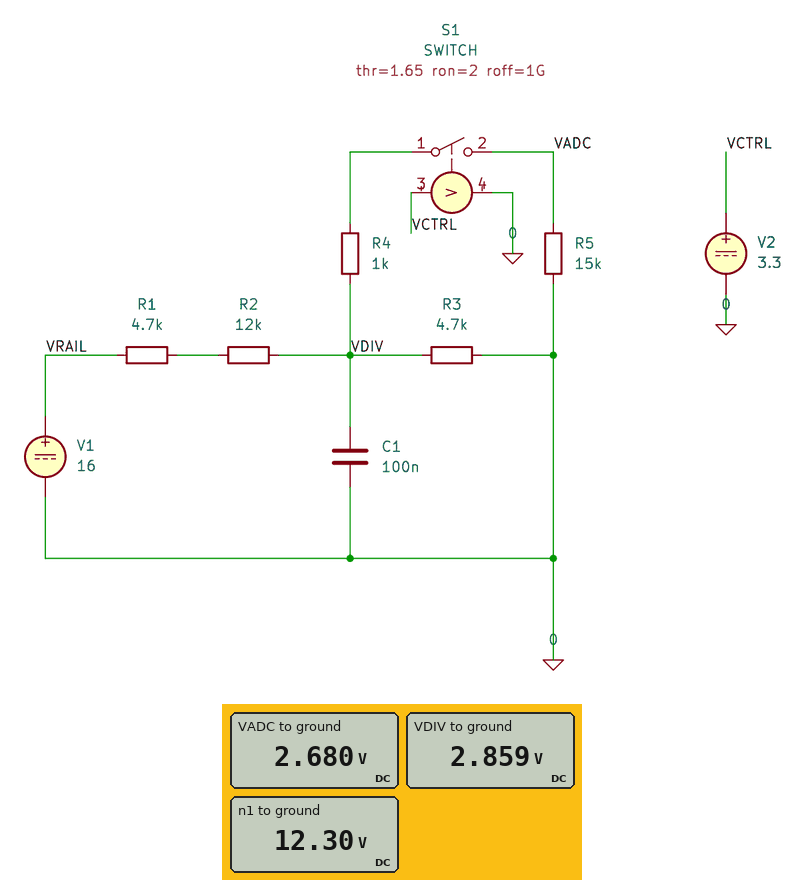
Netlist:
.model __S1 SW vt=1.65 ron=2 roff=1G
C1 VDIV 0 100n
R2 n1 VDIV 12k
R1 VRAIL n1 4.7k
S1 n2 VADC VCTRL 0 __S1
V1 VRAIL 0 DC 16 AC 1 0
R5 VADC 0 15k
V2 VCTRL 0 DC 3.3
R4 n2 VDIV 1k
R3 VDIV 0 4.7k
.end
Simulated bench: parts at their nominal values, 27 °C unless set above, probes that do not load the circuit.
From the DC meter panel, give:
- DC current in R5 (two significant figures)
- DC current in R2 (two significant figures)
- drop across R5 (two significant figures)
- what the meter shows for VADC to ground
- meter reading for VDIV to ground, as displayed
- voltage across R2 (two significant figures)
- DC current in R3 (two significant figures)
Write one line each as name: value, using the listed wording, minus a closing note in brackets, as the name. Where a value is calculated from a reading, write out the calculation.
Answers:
DC current in R5: (2.68 V) / 15 kΩ = 180 µA
DC current in R2: (12.3 V - 2.859 V) / 12 kΩ = 790 µA
drop across R5: 2.68 V = 2.7 V
what the meter shows for VADC to ground: 2.680 V
meter reading for VDIV to ground, as displayed: 2.859 V
voltage across R2: 12.3 V - 2.859 V = 9.4 V
DC current in R3: (2.859 V) / 4.7 kΩ = 610 µA
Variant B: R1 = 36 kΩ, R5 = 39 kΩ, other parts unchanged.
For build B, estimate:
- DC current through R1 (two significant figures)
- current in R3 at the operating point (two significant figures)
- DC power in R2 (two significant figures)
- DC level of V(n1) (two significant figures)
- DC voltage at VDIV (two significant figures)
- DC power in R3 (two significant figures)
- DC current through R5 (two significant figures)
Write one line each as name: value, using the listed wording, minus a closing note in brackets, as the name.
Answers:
DC current through R1: 310 µA
current in R3 at the operating point: 270 µA
DC power in R2: 1.1 mW
DC level of V(n1): 5.0 V
DC voltage at VDIV: 1.3 V
DC power in R3: 350 µW
DC current through R5: 32 µA
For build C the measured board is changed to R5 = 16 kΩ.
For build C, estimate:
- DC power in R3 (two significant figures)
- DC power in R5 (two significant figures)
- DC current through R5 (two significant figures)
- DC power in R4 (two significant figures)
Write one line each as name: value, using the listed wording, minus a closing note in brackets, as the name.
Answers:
DC power in R3: 1.8 mW
DC power in R5: 460 µW
DC current through R5: 170 µA
DC power in R4: 29 µW
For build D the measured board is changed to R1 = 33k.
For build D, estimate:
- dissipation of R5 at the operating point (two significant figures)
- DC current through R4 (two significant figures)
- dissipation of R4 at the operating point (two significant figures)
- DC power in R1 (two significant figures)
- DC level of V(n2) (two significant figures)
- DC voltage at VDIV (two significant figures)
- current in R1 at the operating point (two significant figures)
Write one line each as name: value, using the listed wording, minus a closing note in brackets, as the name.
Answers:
dissipation of R5 at the operating point: 84 µW
DC current through R4: 75 µA
dissipation of R4 at the operating point: 5.6 µW
DC power in R1: 3.6 mW
DC level of V(n2): 1.1 V
DC voltage at VDIV: 1.2 V
current in R1 at the operating point: 330 µA
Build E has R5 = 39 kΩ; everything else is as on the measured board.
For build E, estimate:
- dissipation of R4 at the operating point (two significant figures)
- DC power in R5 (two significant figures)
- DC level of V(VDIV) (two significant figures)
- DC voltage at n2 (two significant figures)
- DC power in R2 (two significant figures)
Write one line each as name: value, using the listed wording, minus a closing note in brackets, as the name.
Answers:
dissipation of R4 at the operating point: 6.5 µW
DC power in R5: 250 µW
DC level of V(VDIV): 3.2 V
DC voltage at n2: 3.1 V
DC power in R2: 7.0 mW
